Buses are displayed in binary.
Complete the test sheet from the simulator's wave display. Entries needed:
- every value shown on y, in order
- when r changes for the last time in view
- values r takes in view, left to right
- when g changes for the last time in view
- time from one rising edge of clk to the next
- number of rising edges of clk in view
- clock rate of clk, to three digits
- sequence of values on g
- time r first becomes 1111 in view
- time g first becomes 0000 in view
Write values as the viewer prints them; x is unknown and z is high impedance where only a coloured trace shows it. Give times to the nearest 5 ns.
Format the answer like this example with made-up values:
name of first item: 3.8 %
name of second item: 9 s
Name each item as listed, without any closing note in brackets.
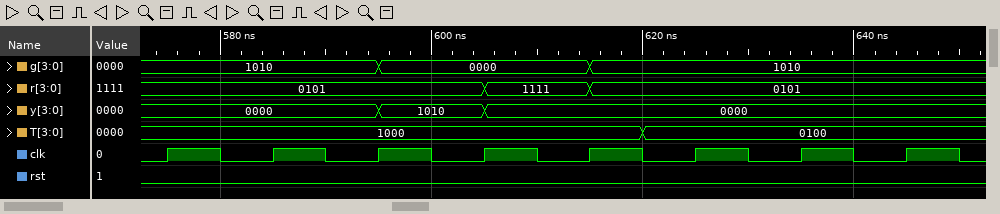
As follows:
every value shown on y, in order: 0000, 1010, 0000
when r changes for the last time in view: 615 ns
values r takes in view, left to right: 0101, 1111, 0101
when g changes for the last time in view: 615 ns
time from one rising edge of clk to the next: 10 ns
number of rising edges of clk in view: 8
clock rate of clk, to three digits: 100 MHz
sequence of values on g: 1010, 0000, 1010
time r first becomes 1111 in view: 605 ns
time g first becomes 0000 in view: 595 ns
